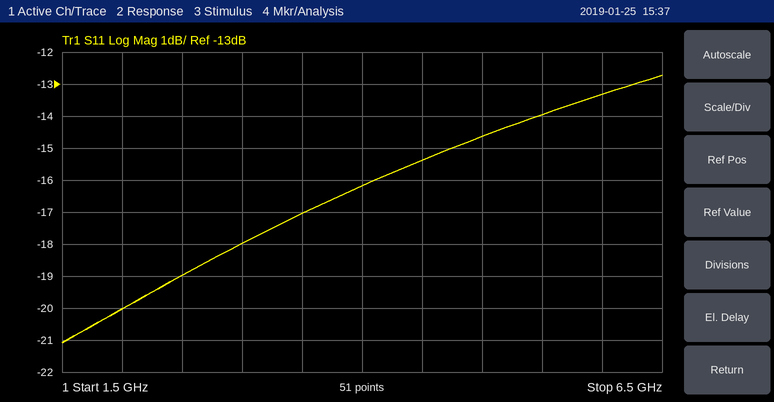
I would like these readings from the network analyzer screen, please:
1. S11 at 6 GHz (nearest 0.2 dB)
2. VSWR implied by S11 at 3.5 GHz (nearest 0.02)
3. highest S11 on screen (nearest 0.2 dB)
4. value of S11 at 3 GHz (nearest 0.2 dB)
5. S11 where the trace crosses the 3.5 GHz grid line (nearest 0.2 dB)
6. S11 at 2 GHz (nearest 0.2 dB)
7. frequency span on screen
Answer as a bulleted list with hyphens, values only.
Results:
- -13.4 dB
- 1.32
- -12.8 dB
- -18.0 dB
- -17.0 dB
- -20.0 dB
- 5 GHz
